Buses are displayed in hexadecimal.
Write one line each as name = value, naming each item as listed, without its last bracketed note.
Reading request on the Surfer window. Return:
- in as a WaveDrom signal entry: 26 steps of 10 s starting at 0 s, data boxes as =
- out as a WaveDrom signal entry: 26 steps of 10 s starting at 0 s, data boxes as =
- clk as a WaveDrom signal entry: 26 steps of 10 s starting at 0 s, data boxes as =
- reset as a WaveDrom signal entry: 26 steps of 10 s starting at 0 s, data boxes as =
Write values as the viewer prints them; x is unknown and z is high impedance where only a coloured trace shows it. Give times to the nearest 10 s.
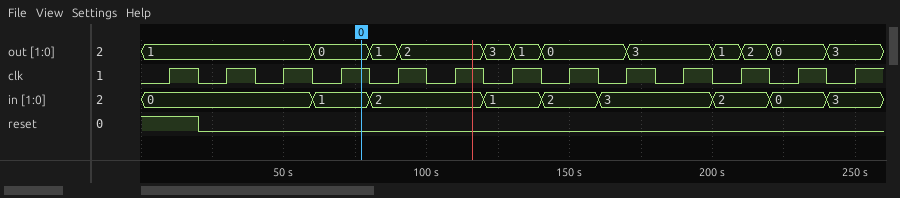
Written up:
in as a WaveDrom signal entry: 26 steps of 10 s starting at 0 s, data boxes as = = {name: 'in', wave: '=.....=.=...=.=.=...=.=.=.', data: '0 1 2 1 2 3 2 0 3'}
out as a WaveDrom signal entry: 26 steps of 10 s starting at 0 s, data boxes as = = {name: 'out', wave: '=.....=.==..===..=..===.=.', data: '1 0 1 2 3 1 0 3 1 2 0 3'}
clk as a WaveDrom signal entry: 26 steps of 10 s starting at 0 s, data boxes as = = {name: 'clk', wave: '01010101010101010101010101'}
reset as a WaveDrom signal entry: 26 steps of 10 s starting at 0 s, data boxes as = = {name: 'reset', wave: '1.0.......................'}
